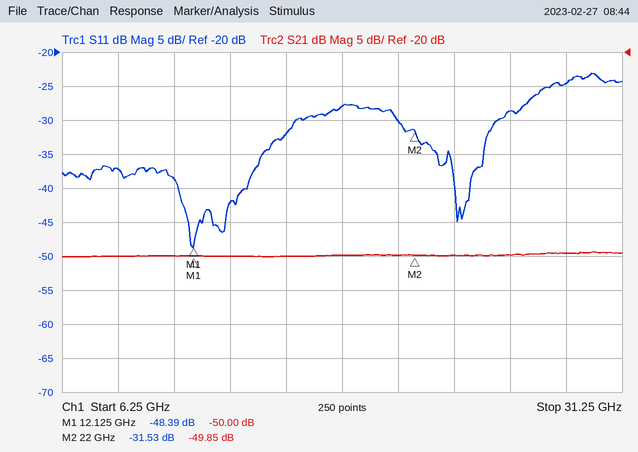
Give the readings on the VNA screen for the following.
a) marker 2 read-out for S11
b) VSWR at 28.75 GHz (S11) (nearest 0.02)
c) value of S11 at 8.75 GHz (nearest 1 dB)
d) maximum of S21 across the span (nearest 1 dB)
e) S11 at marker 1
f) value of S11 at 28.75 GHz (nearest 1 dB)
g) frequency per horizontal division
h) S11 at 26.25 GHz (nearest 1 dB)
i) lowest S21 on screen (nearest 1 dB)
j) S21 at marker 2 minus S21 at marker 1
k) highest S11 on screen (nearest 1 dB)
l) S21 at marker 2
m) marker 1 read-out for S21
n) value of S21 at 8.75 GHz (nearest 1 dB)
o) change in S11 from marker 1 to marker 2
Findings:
-31.53 dB
1.12
-37 dB
-49 dB
-48.39 dB
-25 dB
2.5 GHz
-29 dB
-50 dB
0.15 dB
-23 dB
-49.85 dB
-50.00 dB
-50 dB
16.86 dB
